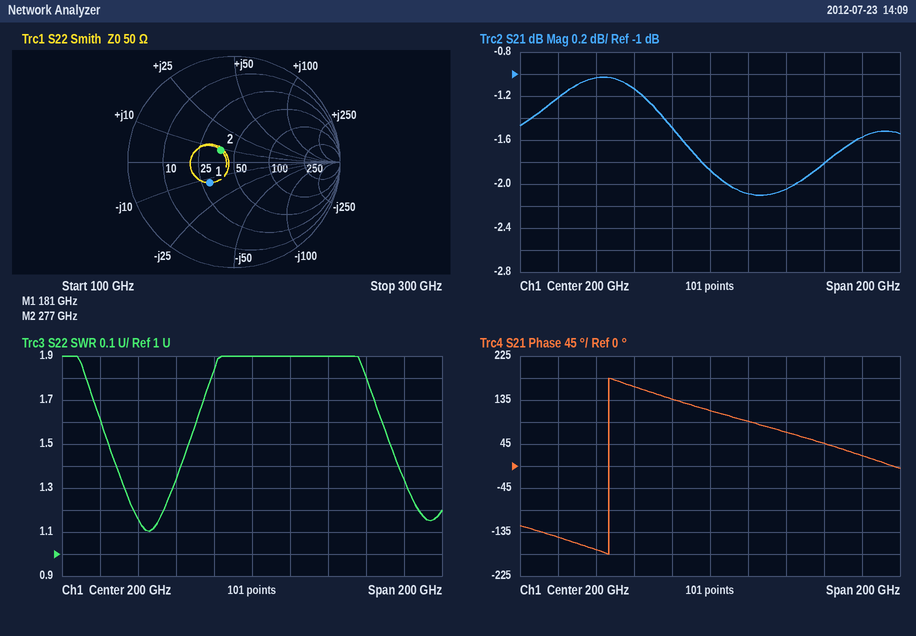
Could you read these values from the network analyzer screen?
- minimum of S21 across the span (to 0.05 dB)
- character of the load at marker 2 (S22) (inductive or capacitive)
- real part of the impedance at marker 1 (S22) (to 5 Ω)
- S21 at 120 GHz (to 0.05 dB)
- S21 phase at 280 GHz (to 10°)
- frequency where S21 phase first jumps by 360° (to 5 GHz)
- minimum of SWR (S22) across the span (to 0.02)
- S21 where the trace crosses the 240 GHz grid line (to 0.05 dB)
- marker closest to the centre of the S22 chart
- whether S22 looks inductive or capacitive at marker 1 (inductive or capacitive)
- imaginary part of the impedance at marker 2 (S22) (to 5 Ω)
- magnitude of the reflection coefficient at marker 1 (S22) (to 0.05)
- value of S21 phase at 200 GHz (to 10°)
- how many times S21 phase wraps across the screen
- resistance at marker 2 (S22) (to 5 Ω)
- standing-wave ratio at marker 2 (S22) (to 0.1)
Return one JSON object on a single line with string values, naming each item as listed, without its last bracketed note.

{"minimum of S21 across the span": "-2.10 dB", "character of the load at marker 2 (S22)": "inductive", "real part of the impedance at marker 1 (S22)": "30 Ω", "S21 at 120 GHz": "-1.20 dB", "S21 phase at 280 GHz": "20°", "frequency where S21 phase first jumps by 360°": "145 GHz", "minimum of SWR (S22) across the span": "1.10", "S21 where the trace crosses the 240 GHz grid line": "-2.05 dB", "marker closest to the centre of the S22 chart": "marker 2", "whether S22 looks inductive or capacitive at marker 1": "capacitive", "imaginary part of the impedance at marker 2 (S22)": "+10 Ω", "magnitude of the reflection coefficient at marker 1 (S22)": "0.30", "value of S21 phase at 200 GHz": "110°", "how many times S21 phase wraps across the screen": "1", "resistance at marker 2 (S22)": "40 Ω", "standing-wave ratio at marker 2 (S22)": "1.4"}
